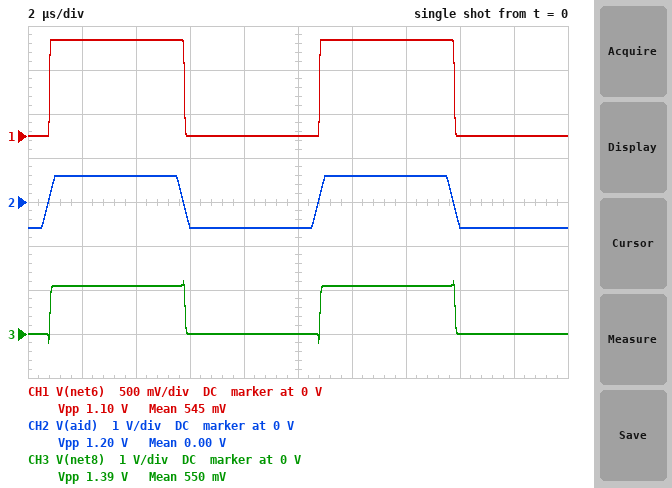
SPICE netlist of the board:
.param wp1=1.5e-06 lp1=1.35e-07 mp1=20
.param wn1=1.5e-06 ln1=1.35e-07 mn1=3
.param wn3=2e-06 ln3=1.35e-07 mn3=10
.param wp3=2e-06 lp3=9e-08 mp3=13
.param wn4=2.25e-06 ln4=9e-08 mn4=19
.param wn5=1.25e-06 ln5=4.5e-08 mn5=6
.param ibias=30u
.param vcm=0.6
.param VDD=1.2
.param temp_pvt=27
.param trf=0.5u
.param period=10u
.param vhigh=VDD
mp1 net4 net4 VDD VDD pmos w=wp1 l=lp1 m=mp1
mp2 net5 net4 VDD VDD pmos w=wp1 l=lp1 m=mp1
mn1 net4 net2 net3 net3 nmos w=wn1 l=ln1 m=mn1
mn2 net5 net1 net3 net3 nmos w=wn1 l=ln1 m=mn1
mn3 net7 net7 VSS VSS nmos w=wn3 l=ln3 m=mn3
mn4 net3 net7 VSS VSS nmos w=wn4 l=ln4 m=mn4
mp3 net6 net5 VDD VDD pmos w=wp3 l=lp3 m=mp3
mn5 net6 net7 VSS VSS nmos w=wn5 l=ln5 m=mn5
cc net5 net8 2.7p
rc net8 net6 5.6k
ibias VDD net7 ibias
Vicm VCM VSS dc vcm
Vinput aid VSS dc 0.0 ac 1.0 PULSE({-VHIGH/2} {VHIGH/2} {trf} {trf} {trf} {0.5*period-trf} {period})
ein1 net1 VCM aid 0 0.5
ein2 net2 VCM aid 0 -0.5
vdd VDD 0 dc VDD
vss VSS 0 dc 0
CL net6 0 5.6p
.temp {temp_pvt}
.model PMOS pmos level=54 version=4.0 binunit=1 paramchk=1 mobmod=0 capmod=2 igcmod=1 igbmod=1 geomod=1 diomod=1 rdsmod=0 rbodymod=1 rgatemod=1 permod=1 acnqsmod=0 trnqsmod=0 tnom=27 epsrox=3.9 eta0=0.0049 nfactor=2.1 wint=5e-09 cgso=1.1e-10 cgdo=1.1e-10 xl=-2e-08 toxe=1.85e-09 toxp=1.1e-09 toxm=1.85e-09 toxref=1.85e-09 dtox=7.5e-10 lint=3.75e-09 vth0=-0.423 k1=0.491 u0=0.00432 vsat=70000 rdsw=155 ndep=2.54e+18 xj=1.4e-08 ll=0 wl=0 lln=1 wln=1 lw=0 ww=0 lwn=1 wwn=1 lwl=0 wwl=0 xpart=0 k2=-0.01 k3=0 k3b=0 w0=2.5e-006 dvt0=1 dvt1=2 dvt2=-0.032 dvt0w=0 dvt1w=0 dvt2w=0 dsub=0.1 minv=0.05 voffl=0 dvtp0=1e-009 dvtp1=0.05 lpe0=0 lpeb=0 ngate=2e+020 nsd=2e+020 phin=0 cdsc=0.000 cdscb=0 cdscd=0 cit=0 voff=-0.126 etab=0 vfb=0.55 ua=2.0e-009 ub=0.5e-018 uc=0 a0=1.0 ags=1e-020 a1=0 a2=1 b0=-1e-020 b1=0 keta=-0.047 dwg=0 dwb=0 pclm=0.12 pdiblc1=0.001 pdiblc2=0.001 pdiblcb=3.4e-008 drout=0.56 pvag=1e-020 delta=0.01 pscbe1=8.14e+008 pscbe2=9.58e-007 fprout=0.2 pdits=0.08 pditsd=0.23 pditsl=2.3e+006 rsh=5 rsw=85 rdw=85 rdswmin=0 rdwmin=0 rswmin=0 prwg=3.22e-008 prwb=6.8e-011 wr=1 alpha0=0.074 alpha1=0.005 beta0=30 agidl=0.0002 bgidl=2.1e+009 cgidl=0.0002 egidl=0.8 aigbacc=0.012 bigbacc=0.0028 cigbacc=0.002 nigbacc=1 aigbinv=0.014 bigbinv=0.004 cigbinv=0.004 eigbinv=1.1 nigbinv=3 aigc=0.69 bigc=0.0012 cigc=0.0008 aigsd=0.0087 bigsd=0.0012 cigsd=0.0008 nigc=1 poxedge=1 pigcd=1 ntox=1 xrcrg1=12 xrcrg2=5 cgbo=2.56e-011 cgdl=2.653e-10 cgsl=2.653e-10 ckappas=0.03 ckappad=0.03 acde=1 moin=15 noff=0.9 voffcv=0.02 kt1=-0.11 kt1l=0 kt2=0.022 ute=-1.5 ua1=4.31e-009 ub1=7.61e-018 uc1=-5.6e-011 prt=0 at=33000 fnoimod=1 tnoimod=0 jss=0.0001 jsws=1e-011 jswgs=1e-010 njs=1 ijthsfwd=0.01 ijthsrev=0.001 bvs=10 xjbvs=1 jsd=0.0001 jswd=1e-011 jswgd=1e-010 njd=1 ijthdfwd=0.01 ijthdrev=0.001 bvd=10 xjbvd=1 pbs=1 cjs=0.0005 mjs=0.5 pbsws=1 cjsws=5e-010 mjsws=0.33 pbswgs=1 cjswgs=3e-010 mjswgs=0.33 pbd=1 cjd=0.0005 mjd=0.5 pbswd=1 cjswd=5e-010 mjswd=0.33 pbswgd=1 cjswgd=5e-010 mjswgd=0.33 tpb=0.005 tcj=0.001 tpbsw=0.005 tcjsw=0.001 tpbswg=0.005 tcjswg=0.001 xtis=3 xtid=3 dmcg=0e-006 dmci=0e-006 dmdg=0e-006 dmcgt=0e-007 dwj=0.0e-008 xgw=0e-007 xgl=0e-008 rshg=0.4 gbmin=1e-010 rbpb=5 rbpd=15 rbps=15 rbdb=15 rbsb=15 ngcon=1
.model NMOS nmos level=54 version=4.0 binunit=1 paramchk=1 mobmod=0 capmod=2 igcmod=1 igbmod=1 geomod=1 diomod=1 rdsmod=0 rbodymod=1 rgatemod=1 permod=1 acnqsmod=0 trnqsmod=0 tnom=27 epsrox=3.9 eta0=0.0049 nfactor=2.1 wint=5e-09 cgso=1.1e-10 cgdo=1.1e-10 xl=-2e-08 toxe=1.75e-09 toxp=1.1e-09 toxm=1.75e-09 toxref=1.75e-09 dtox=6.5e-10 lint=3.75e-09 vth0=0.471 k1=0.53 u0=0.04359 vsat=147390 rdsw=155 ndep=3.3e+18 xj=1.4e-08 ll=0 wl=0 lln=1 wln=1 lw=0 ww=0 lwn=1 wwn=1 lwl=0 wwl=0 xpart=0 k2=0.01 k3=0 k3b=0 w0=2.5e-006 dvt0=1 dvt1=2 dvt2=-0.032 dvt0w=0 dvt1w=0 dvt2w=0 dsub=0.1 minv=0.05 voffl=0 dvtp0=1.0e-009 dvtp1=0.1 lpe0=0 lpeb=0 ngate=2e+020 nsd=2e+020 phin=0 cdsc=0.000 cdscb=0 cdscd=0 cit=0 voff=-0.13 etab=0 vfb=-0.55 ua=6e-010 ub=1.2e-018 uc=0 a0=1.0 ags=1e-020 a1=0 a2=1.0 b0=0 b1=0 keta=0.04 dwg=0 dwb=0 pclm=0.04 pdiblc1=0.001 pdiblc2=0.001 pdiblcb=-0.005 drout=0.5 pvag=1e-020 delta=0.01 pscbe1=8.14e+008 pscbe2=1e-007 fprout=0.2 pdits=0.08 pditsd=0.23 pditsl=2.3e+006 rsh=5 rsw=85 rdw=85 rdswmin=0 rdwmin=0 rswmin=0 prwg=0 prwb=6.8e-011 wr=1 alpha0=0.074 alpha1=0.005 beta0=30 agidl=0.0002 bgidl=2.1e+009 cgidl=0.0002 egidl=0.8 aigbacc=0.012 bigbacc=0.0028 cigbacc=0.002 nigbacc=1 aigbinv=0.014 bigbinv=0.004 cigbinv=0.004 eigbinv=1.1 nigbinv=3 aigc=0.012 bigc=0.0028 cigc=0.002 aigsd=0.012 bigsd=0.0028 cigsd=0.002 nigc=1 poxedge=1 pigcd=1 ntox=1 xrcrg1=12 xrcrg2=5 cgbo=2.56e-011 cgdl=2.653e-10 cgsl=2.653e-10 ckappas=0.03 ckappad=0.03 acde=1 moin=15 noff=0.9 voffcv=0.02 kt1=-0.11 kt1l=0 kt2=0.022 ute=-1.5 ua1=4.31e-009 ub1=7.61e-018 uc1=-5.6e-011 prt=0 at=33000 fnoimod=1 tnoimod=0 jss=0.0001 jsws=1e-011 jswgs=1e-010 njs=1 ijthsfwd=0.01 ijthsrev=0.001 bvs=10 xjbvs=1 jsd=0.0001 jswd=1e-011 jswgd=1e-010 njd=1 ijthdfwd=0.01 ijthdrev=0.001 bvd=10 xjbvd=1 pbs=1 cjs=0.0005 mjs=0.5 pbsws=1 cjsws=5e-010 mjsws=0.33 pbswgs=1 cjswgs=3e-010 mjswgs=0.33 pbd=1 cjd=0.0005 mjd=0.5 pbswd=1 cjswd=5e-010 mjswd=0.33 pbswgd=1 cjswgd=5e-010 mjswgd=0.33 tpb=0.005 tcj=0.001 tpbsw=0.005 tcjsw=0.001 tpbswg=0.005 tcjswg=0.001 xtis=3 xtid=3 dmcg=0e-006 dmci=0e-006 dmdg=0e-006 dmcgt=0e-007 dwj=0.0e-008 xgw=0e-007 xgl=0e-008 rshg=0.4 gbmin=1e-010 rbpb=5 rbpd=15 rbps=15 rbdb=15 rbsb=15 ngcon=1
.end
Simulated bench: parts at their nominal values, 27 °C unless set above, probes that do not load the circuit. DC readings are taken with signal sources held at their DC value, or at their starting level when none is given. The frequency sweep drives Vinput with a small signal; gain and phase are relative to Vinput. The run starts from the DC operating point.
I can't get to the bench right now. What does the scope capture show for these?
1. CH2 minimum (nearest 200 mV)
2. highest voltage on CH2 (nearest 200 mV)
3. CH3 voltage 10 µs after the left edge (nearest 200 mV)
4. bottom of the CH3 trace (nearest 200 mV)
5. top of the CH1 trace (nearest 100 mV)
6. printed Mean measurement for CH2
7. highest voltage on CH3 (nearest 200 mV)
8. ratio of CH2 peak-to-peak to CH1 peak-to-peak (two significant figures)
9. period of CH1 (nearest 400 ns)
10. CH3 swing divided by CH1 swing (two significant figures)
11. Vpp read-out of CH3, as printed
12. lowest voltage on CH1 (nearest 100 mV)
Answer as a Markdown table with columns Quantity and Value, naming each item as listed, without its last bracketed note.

| Quantity | Value |
|---|---|
| CH2 minimum | -600 mV |
| highest voltage on CH2 | 600 mV |
| CH3 voltage 10 µs after the left edge | 0 V |
| bottom of the CH3 trace | -200 mV |
| top of the CH1 trace | 1.1 V |
| printed Mean measurement for CH2 | 0.00 V |
| highest voltage on CH3 | 1.2 V |
| ratio of CH2 peak-to-peak to CH1 peak-to-peak | 1.1 |
| period of CH1 | 10.0 µs |
| CH3 swing divided by CH1 swing | 1.3 |
| Vpp read-out of CH3, as printed | 1.39 V |
| lowest voltage on CH1 | 0 V |
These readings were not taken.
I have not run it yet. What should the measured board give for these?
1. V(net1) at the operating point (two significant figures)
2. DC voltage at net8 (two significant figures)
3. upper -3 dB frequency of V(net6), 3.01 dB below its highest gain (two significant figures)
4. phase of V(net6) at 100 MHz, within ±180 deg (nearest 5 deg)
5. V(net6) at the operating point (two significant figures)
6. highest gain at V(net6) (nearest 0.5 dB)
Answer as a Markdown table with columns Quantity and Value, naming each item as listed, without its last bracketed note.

| Quantity | Value |
|---|---|
| V(net1) at the operating point | 600 mV |
| DC voltage at net8 | 150 mV |
| upper -3 dB frequency of V(net6), 3.01 dB below its highest gain | 170 kHz |
| phase of V(net6) at 100 MHz, within ±180 deg | -90 deg |
| V(net6) at the operating point | 150 mV |
| highest gain at V(net6) | 47.0 dB |
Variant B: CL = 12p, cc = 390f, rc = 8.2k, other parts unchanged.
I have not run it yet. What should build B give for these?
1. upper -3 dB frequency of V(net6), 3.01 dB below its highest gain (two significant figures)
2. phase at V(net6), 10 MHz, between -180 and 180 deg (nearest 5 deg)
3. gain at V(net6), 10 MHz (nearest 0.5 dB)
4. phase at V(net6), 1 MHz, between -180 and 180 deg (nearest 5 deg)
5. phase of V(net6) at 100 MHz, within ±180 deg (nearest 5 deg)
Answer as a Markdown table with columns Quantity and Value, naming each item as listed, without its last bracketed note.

| Quantity | Value |
|---|---|
| upper -3 dB frequency of V(net6), 3.01 dB below its highest gain | 940 kHz |
| phase at V(net6), 10 MHz, between -180 and 180 deg | -100 deg |
| gain at V(net6), 10 MHz | 26.0 dB |
| phase at V(net6), 1 MHz, between -180 and 180 deg | -50 deg |
| phase of V(net6) at 100 MHz, within ±180 deg | -125 deg |
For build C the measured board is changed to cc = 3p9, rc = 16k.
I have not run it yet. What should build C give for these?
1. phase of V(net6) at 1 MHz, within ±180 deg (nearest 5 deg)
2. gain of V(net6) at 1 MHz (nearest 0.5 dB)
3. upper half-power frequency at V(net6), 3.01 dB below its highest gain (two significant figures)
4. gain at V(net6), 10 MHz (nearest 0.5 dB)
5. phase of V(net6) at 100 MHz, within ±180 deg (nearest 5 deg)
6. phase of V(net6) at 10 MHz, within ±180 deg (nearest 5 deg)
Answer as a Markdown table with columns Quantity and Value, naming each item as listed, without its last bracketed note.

| Quantity | Value |
|---|---|
| phase of V(net6) at 1 MHz, within ±180 deg | -65 deg |
| gain of V(net6) at 1 MHz | 28.5 dB |
| upper half-power frequency at V(net6), 3.01 dB below its highest gain | 110 kHz |
| gain at V(net6), 10 MHz | 19.5 dB |
| phase of V(net6) at 100 MHz, within ±180 deg | -105 deg |
| phase of V(net6) at 10 MHz, within ±180 deg | -30 deg |
